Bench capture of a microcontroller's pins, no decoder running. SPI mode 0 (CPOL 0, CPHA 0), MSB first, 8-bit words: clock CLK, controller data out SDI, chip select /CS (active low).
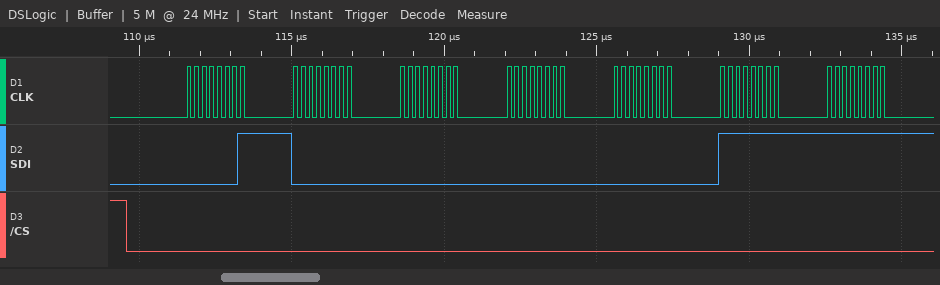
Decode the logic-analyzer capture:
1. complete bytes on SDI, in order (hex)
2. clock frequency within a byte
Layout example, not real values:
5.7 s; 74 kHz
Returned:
01 00 00 00 00 FF FF; 4 MHz
